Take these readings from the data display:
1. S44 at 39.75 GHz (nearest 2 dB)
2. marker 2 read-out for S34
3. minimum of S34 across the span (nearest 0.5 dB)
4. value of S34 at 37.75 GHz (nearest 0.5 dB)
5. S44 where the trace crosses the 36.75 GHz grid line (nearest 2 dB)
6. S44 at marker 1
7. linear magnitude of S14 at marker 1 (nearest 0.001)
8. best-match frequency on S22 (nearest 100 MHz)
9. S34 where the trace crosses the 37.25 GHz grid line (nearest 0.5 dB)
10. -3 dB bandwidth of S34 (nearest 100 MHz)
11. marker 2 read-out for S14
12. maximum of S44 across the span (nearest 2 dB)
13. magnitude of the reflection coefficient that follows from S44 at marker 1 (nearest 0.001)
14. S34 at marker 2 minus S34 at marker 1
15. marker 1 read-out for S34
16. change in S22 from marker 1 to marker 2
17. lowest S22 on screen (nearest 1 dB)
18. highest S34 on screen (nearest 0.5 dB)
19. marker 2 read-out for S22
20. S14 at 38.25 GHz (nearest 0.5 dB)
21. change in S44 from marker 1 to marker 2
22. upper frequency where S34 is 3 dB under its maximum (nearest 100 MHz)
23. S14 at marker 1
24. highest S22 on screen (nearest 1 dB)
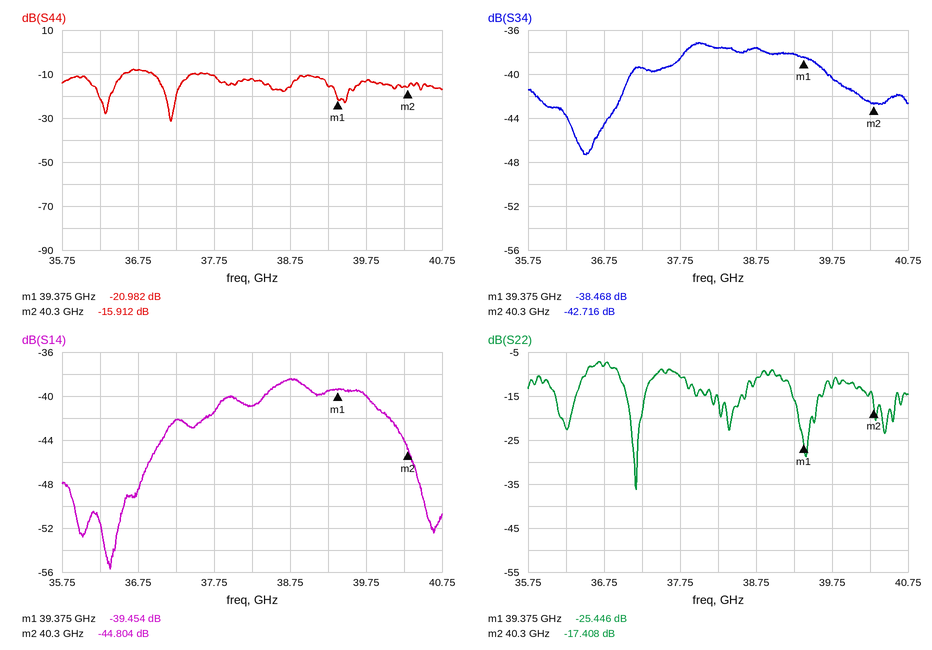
-14 dB
-42.716 dB
-47.5 dB
-38.5 dB
-8 dB
-20.982 dB
0.011
37.2 GHz
-39.5 dB
2.6 GHz
-44.804 dB
-8 dB
0.089
-4.248 dB
-38.468 dB
8.038 dB
-36 dB
-37.0 dB
-17.408 dB
-41.0 dB
5.070 dB
39.7 GHz
-39.454 dB
-7 dB
